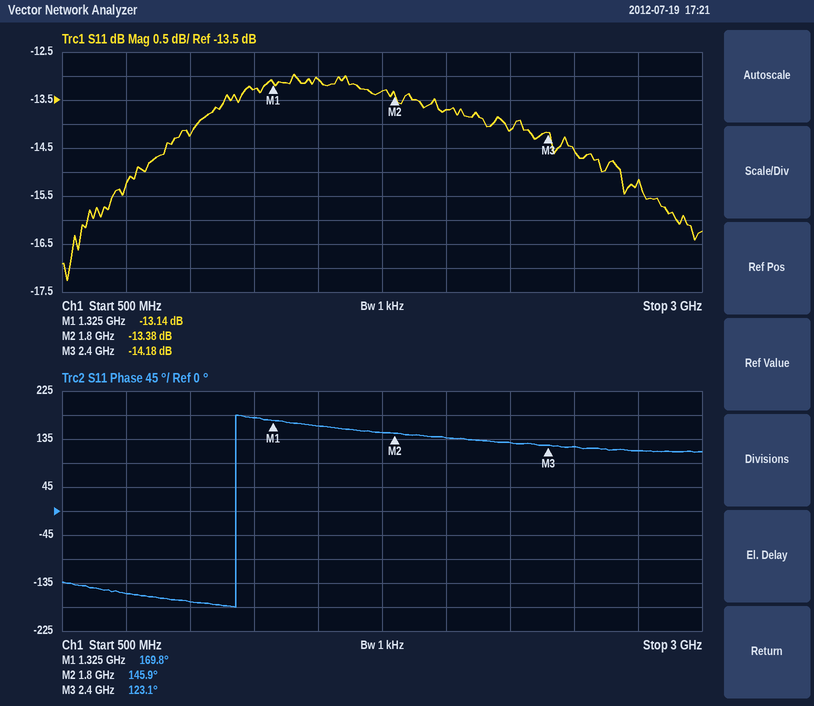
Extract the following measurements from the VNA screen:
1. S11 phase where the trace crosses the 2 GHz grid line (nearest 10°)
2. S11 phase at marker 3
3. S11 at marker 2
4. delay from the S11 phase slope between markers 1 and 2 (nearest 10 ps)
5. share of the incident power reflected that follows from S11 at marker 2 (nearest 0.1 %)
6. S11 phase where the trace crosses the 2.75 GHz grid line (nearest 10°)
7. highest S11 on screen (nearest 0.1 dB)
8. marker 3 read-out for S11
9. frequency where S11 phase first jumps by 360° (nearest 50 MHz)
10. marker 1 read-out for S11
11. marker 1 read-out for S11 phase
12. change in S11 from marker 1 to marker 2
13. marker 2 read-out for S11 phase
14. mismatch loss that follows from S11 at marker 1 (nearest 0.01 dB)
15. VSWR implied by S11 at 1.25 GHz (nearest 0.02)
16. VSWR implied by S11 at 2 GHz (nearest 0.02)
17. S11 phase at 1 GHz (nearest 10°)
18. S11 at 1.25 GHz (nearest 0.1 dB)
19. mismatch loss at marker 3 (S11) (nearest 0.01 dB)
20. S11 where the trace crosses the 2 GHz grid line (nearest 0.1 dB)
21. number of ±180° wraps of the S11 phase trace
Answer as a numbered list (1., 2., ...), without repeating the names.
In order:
1. 140°
2. 123.1°
3. -13.38 dB
4. 140 ps
5. 4.6 %
6. 110°
7. -13.0 dB
8. -14.18 dB
9. 1.20 GHz
10. -13.14 dB
11. 169.8°
12. -0.24 dB
13. 145.9°
14. 0.22 dB
15. 1.56
16. 1.52
17. -170°
18. -13.3 dB
19. 0.17 dB
20. -13.7 dB
21. 1
